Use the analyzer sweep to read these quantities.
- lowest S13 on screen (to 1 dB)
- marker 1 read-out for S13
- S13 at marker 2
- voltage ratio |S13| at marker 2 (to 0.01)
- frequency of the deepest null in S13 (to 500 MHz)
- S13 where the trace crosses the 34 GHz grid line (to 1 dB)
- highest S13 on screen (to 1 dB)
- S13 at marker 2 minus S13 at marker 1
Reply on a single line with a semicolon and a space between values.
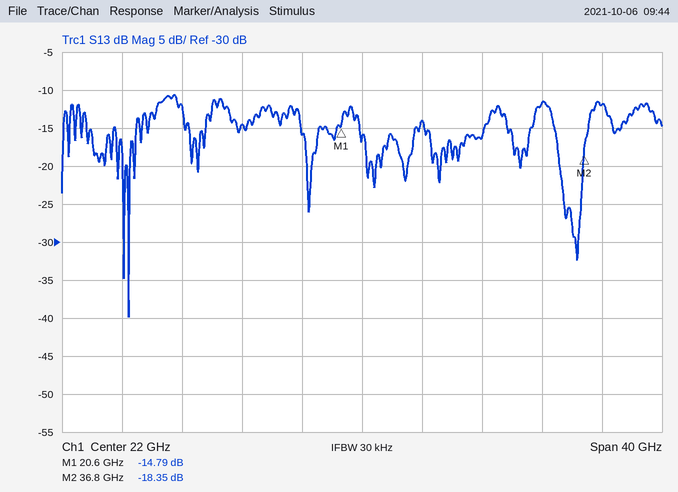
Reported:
-40 dB; -14.79 dB; -18.35 dB; 0.12; 6.5 GHz; -12 dB; -11 dB; -3.56 dB
